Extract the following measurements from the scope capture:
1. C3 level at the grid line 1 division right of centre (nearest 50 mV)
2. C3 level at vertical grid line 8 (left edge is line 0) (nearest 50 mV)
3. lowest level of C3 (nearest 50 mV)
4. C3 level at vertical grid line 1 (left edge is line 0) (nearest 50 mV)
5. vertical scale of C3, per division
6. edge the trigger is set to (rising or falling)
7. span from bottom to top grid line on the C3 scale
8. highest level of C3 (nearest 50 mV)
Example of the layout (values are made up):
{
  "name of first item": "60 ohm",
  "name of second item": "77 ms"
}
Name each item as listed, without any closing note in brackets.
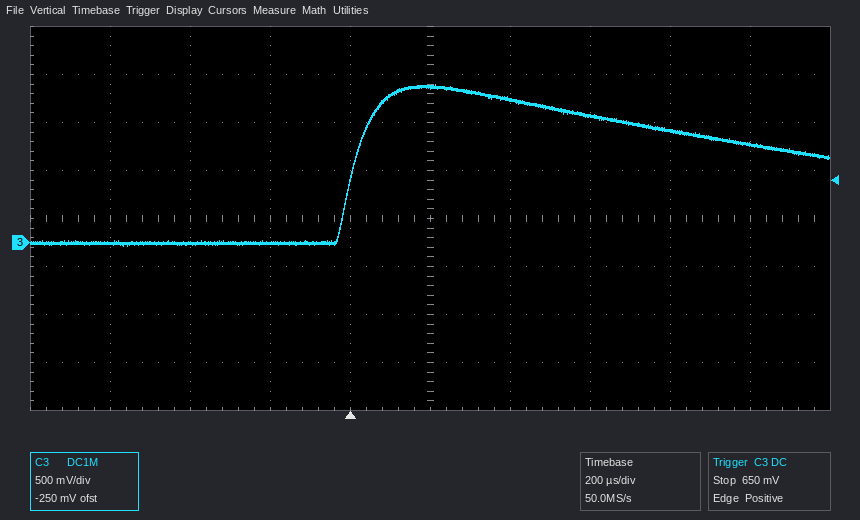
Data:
{
  "C3 level at the grid line 1 division right of centre": "1.50 V",
  "C3 level at vertical grid line 8 (left edge is line 0)": "1.15 V",
  "lowest level of C3": "-50 mV",
  "C3 level at vertical grid line 1 (left edge is line 0)": "0 mV",
  "vertical scale of C3, per division": "500 mV",
  "edge the trigger is set to": "rising",
  "span from bottom to top grid line on the C3 scale": "4 V",
  "highest level of C3": "1.65 V"
}
